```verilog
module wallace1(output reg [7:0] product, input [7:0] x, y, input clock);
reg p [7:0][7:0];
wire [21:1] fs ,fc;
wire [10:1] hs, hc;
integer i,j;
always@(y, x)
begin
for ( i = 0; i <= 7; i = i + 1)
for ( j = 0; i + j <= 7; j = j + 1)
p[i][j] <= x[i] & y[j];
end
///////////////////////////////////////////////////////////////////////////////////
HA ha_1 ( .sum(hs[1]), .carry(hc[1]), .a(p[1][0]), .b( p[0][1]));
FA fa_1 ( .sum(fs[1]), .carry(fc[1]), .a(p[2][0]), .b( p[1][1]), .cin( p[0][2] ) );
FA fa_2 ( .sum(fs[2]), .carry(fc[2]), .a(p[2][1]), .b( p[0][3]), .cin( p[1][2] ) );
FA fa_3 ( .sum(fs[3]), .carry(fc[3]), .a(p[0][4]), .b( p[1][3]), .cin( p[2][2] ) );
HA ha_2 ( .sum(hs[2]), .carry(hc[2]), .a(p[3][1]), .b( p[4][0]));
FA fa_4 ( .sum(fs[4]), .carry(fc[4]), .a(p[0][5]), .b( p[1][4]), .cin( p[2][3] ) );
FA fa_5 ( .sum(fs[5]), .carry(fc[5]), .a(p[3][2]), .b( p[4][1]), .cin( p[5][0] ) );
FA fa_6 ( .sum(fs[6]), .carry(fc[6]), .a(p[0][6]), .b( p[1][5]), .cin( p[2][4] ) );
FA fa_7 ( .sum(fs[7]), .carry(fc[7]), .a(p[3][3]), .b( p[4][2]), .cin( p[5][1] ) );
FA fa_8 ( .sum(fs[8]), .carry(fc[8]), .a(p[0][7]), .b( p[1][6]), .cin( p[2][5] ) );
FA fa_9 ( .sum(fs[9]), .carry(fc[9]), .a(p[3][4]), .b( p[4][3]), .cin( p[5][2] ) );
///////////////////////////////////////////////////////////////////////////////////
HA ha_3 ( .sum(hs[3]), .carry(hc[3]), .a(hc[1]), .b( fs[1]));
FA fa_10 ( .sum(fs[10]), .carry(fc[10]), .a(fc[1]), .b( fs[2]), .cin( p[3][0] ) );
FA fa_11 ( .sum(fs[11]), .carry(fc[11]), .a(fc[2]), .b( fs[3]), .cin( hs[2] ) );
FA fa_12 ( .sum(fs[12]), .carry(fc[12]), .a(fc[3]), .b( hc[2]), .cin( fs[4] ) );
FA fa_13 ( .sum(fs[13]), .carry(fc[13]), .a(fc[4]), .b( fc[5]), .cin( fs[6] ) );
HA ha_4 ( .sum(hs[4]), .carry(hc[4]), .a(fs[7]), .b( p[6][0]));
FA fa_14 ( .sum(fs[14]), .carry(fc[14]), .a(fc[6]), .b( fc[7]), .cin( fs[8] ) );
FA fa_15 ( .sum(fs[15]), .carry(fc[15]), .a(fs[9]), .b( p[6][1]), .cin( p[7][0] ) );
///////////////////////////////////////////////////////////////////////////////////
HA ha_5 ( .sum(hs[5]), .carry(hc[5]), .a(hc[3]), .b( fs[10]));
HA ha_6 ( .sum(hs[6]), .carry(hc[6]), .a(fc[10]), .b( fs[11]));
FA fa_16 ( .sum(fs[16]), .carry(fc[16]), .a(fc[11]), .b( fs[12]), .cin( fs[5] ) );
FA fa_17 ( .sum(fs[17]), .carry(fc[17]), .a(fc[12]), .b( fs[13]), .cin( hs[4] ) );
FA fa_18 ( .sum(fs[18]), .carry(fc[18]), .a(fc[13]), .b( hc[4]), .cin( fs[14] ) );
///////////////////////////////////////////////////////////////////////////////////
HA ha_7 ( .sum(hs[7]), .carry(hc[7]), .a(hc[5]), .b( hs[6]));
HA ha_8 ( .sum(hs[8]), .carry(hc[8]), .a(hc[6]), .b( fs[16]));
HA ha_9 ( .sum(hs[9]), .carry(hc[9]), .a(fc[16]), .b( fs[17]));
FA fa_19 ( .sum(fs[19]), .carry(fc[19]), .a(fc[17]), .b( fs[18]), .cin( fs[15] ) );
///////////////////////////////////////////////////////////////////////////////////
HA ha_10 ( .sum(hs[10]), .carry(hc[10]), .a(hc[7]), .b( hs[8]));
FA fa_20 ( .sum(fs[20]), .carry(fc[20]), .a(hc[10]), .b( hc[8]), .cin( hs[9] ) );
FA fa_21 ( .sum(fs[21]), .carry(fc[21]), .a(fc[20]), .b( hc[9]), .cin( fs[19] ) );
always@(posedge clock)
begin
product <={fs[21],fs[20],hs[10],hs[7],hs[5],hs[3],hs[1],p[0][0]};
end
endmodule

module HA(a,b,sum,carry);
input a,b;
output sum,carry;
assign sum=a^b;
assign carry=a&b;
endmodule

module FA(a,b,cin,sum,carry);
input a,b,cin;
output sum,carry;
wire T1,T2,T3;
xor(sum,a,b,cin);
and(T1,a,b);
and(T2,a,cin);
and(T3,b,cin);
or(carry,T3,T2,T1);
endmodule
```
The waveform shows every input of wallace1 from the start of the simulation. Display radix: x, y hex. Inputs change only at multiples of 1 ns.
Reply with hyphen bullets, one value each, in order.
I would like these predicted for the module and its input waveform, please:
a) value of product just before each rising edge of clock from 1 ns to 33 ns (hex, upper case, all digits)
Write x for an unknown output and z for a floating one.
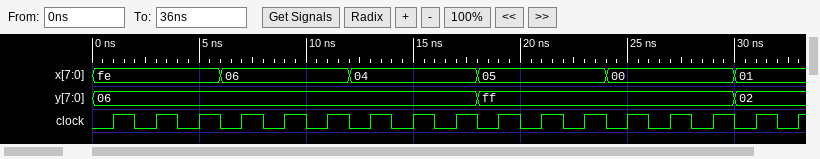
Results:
- x, F4, F4, F4, 24, 24, 24, 18, 18, 18, FB, FB, FB, 00, 00, 00, 02
